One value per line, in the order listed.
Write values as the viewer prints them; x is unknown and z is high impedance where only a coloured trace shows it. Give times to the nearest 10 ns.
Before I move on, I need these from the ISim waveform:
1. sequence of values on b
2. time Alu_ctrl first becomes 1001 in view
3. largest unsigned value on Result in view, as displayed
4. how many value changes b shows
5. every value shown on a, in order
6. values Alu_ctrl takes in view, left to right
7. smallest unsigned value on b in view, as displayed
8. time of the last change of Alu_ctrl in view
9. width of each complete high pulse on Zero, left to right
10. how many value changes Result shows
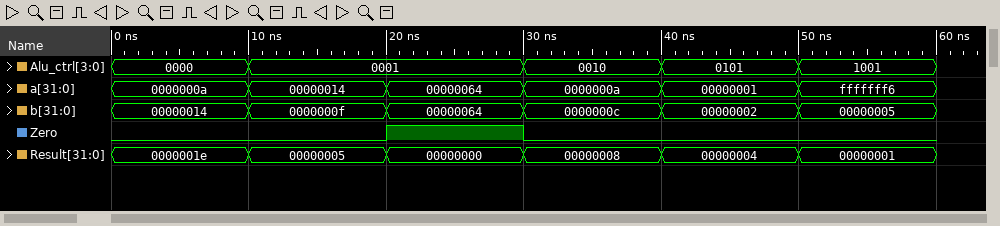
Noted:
00000014, 0000000f, 00000064, 0000000c, 00000002, 00000005
50 ns
0000001e
5
0000000a, 00000014, 00000064, 0000000a, 00000001, fffffff6
0000, 0001, 0010, 0101, 1001
00000002
50 ns
10 ns
5
